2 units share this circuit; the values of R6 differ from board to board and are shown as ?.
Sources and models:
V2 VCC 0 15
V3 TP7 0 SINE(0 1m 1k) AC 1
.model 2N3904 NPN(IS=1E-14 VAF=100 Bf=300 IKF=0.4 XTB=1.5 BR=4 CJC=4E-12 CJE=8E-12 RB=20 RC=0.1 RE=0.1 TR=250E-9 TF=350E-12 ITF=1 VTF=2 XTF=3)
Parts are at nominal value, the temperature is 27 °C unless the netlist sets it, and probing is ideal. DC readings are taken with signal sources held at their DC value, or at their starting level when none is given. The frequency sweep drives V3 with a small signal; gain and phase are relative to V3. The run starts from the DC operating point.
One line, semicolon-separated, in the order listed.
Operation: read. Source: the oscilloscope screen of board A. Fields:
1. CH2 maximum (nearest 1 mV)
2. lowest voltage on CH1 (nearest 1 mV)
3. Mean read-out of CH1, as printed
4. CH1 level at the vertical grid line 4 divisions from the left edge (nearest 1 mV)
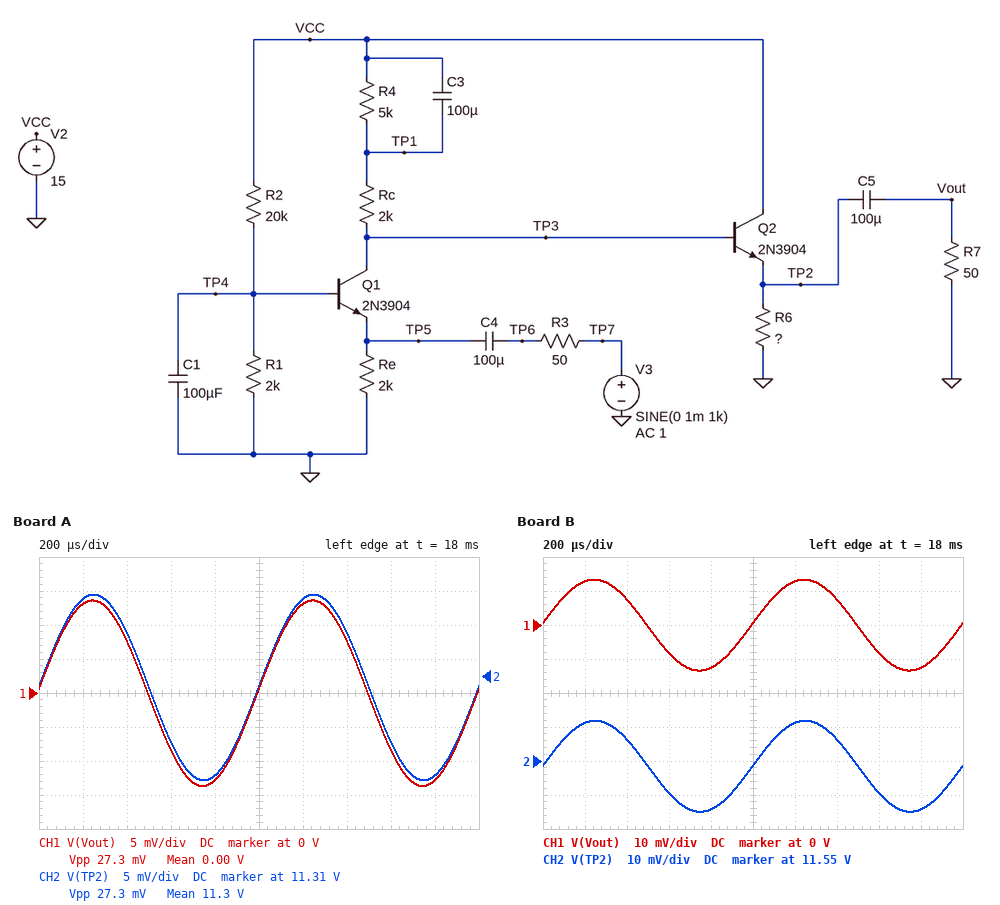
11.327 V; -14 mV; 0.00 V; -13 mV
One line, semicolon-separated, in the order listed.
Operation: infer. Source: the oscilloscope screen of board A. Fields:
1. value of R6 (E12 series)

680 Ω
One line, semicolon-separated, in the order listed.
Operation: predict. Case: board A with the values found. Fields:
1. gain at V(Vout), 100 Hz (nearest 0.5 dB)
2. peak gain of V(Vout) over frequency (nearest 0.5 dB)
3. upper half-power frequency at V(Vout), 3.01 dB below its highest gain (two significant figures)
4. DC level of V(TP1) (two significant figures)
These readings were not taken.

22.5 dB; 22.5 dB; 7.5 MHz; 13 V
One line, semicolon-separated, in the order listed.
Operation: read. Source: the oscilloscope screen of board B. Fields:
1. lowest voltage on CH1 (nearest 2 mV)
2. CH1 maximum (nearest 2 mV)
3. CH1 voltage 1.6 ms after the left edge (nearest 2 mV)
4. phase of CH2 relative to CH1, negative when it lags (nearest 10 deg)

-14 mV; 14 mV; -8 mV; 0 deg
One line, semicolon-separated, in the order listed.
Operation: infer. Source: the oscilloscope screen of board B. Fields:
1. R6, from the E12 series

1.5 kΩ
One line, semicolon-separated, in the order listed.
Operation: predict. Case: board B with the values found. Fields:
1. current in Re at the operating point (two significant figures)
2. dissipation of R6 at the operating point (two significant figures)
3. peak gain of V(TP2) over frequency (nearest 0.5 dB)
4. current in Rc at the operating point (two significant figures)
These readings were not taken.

370 µA; 89 mW; 22.5 dB; 390 µA
